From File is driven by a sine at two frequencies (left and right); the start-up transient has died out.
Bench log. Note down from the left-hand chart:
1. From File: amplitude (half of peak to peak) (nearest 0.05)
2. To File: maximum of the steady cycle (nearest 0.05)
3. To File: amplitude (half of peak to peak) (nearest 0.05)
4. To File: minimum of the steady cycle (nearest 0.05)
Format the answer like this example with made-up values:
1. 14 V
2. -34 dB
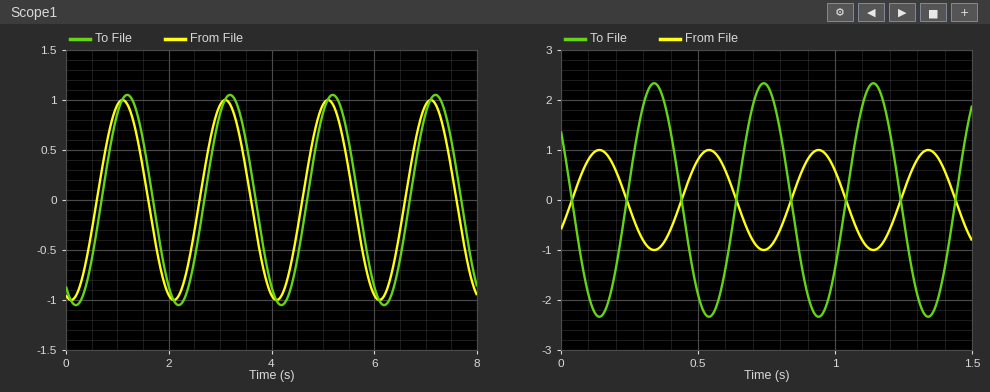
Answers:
1. 1.00
2. 1.05
3. 1.05
4. -1.05
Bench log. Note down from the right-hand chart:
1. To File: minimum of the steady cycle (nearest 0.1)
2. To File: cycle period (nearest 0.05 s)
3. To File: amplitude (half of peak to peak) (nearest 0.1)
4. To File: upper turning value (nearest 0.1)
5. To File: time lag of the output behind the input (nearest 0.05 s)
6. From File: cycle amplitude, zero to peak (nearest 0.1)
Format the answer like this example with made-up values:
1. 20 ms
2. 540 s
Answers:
1. -2.3
2. 0.40 s
3. 2.3
4. 2.3
5. 0.20 s
6. 1.0
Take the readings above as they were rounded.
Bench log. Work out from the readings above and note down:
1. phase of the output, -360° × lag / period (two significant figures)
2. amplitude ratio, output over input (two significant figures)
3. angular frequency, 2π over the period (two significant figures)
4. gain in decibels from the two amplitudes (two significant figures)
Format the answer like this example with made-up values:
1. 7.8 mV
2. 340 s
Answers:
1. -180°
2. 2.3
3. 16 rad/s
4. 7.2 dB
